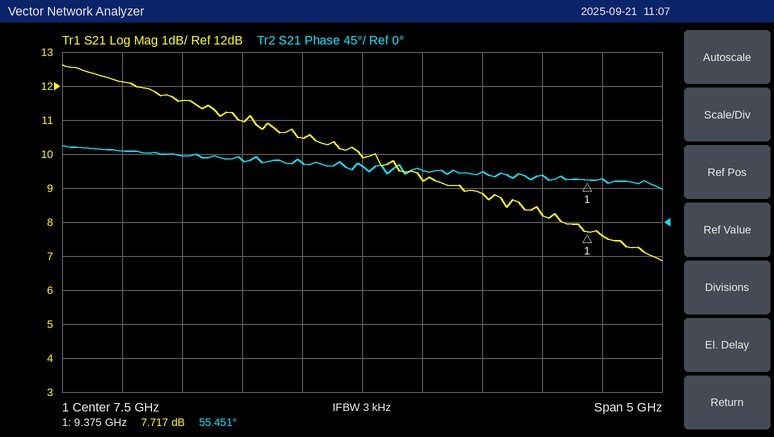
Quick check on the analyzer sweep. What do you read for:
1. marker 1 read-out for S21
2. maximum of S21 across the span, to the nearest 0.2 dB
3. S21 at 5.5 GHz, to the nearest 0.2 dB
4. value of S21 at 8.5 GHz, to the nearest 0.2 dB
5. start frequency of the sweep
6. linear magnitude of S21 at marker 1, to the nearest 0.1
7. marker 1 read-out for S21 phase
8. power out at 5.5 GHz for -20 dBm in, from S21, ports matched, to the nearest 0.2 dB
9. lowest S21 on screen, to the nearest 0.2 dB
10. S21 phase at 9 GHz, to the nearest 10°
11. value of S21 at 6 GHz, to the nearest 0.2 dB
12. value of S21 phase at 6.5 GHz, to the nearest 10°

7.717 dB
12.6 dB
12.2 dB
8.8 dB
5 GHz
2.4
55.451°
-7.8 dBm
6.8 dB
60°
11.6 dB
80°
